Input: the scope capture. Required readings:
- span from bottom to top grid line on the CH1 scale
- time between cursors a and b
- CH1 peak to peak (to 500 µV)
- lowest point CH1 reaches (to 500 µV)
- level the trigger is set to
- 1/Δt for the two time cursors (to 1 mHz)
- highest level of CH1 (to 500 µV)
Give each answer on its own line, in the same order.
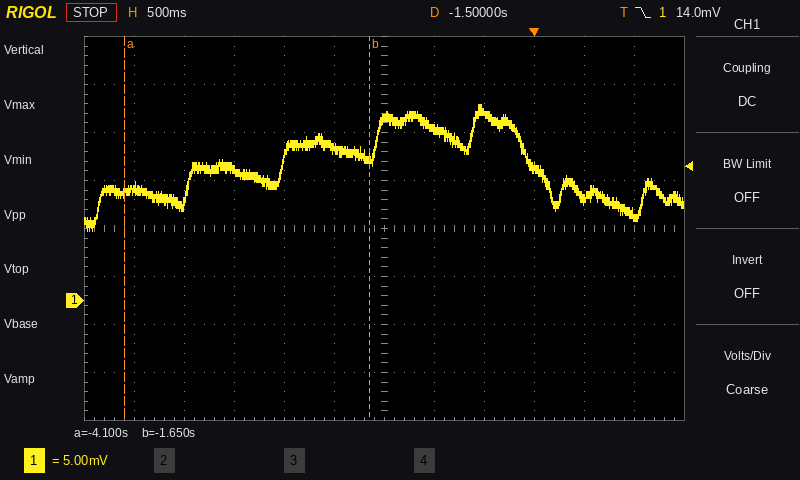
40 mV
2.45 s
13.0 mV
7.5 mV
14.0 mV
408 mHz
20.5 mV
